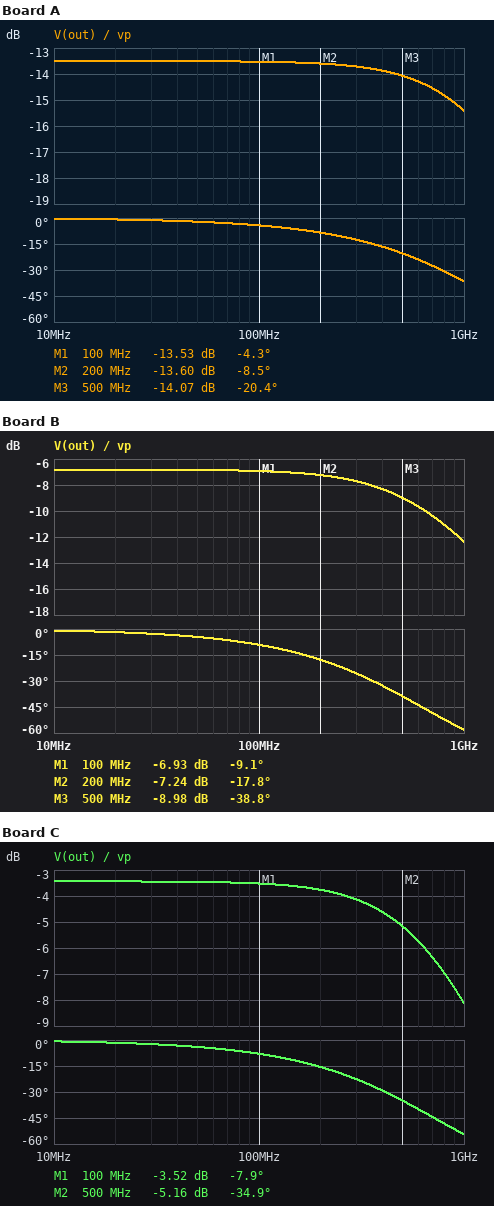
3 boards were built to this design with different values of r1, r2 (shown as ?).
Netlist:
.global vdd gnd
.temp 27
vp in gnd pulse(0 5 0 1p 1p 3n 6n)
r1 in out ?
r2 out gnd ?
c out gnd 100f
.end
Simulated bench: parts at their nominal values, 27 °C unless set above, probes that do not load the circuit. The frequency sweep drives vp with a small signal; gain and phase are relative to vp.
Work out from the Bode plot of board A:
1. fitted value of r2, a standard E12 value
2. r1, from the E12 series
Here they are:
1.5 kΩ
5.6 kΩ
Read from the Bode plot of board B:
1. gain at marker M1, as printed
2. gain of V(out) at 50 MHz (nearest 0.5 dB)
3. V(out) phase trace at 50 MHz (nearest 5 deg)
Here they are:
-6.93 dB
-7.0 dB
-5 deg
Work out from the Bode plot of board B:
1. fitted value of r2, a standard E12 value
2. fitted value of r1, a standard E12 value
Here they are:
4.7 kΩ
5.6 kΩ
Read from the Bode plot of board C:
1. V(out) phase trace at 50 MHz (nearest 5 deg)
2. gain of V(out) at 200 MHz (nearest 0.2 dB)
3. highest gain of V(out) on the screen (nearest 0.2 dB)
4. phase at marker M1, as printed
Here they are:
-5 deg
-3.8 dB
-3.4 dB
-7.9 deg
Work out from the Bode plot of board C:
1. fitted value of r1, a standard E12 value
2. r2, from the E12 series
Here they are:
3.3 kΩ
6.8 kΩ
